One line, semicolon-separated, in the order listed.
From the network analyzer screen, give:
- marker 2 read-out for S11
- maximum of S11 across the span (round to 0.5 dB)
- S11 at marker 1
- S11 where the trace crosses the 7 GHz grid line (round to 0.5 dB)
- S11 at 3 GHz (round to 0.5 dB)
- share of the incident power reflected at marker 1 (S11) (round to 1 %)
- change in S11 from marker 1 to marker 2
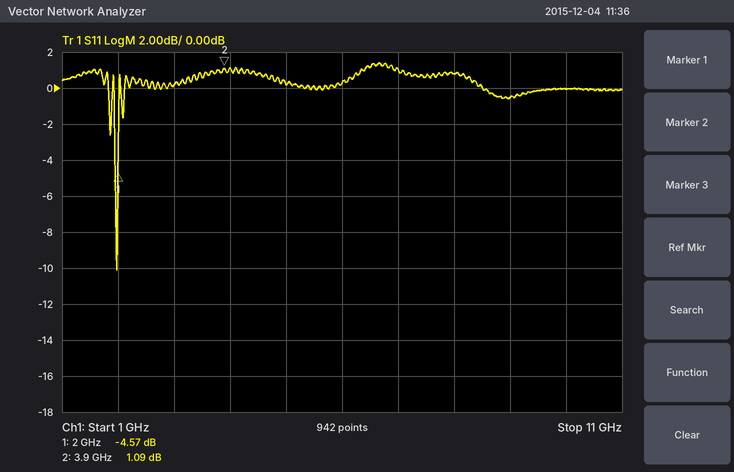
1.09 dB; 1.5 dB; -4.57 dB; 1.0 dB; 0.0 dB; 35 %; 5.66 dB
